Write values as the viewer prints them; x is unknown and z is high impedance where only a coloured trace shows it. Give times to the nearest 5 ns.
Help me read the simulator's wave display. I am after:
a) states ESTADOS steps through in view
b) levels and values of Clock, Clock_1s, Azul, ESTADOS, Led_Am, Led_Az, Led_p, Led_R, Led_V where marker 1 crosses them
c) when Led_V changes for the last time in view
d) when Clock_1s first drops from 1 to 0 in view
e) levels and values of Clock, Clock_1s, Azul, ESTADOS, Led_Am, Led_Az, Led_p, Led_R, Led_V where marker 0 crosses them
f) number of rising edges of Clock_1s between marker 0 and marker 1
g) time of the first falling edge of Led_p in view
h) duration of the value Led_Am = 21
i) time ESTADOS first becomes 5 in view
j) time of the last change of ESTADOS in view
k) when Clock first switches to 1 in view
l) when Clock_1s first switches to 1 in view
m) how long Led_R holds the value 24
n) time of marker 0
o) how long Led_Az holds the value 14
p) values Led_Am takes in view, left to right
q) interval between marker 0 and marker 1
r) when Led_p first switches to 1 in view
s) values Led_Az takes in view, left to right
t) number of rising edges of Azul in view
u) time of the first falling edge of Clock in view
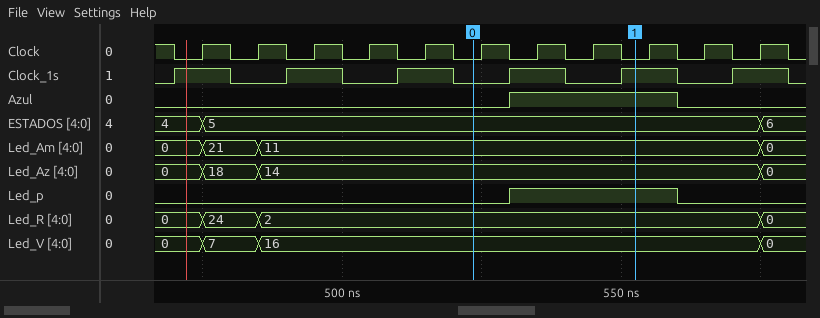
4, 5, 6
Clock=0, Clock_1s=1, Azul=1, ESTADOS=5, Led_Am=11, Led_Az=14, Led_p=1, Led_R=2, Led_V=16
575 ns
480 ns
Clock=0, Clock_1s=0, Azul=0, ESTADOS=5, Led_Am=11, Led_Az=14, Led_p=0, Led_R=2, Led_V=16
2
560 ns
10 ns
475 ns
575 ns
475 ns
470 ns
10 ns
525 ns
90 ns
0, 21, 11, 0
30 ns
530 ns
0, 18, 14, 0
1
470 ns
